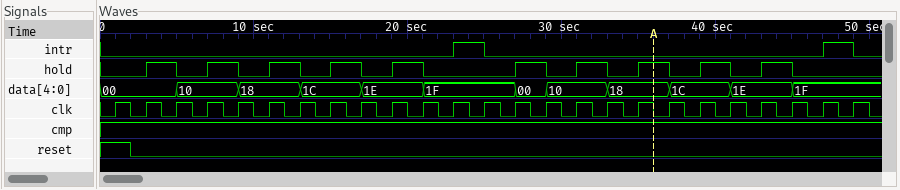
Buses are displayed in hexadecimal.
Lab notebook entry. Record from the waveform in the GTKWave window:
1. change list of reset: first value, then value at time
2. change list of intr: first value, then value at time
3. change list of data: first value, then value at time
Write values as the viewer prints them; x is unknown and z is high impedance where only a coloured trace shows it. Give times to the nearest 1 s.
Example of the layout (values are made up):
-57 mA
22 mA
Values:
1, 0 at 2 s
0, 1 at 23 s, 0 at 25 s, 1 at 47 s, 0 at 49 s
00, 10 at 5 s, 18 at 9 s, 1C at 13 s, 1E at 17 s, 1F at 21 s, 00 at 27 s, 10 at 29 s, 18 at 33 s, 1C at 37 s, 1E at 41 s, 1F at 45 s
